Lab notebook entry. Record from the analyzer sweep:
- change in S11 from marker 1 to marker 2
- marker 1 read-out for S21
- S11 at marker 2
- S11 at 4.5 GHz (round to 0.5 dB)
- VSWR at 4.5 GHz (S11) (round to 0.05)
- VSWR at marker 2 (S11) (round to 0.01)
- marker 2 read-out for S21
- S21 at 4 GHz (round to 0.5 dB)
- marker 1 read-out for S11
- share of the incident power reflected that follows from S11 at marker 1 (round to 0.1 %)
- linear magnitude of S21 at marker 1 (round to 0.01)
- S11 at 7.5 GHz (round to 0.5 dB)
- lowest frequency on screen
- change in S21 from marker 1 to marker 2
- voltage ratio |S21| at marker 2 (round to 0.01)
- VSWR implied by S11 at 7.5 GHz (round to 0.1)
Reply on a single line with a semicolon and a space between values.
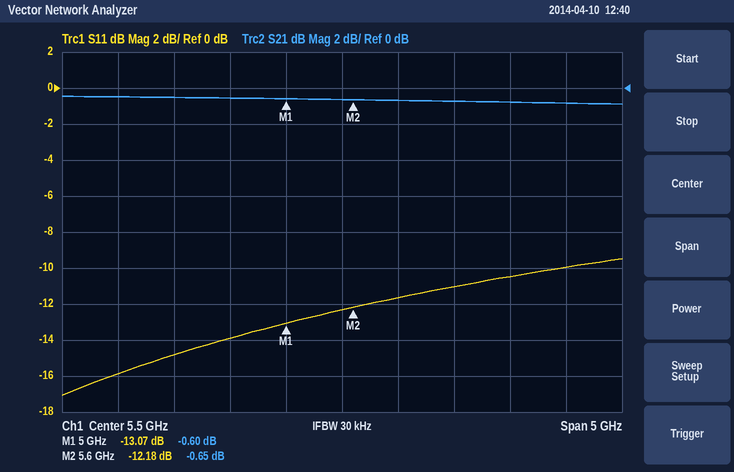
0.89 dB; -0.60 dB; -12.18 dB; -14.0 dB; 1.50; 1.65; -0.65 dB; -0.5 dB; -13.07 dB; 4.9 %; 0.93; -10.0 dB; 3 GHz; -0.05 dB; 0.93; 1.9
